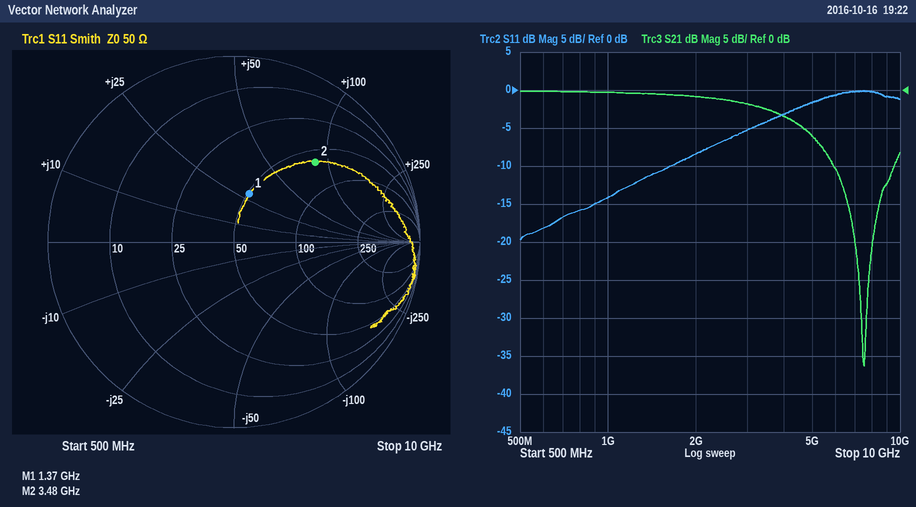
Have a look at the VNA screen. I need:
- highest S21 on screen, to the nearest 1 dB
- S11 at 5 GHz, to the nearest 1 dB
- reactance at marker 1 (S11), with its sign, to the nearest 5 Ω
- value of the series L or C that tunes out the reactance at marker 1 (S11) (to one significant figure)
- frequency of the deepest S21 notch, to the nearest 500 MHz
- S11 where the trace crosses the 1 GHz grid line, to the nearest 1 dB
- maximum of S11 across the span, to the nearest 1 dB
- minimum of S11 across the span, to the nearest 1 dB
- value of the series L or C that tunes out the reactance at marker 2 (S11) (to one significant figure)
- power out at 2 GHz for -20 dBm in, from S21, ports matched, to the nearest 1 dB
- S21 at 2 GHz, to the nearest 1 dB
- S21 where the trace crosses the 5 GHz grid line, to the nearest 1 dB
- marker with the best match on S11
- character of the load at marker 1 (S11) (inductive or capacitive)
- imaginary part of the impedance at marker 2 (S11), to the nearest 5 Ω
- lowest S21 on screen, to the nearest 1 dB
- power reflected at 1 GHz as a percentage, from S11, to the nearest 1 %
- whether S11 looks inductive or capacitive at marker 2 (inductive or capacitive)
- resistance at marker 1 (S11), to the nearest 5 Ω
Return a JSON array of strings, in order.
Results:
["0 dB", "-2 dB", "+30 Ω", "4 pF", "7.5 GHz", "-14 dB", "0 dB", "-20 dB", "500 fF", "-21 dBm", "-1 dB", "-6 dB", "marker 1", "inductive", "+85 Ω", "-36 dB", "4 %", "inductive", "50 Ω"]
